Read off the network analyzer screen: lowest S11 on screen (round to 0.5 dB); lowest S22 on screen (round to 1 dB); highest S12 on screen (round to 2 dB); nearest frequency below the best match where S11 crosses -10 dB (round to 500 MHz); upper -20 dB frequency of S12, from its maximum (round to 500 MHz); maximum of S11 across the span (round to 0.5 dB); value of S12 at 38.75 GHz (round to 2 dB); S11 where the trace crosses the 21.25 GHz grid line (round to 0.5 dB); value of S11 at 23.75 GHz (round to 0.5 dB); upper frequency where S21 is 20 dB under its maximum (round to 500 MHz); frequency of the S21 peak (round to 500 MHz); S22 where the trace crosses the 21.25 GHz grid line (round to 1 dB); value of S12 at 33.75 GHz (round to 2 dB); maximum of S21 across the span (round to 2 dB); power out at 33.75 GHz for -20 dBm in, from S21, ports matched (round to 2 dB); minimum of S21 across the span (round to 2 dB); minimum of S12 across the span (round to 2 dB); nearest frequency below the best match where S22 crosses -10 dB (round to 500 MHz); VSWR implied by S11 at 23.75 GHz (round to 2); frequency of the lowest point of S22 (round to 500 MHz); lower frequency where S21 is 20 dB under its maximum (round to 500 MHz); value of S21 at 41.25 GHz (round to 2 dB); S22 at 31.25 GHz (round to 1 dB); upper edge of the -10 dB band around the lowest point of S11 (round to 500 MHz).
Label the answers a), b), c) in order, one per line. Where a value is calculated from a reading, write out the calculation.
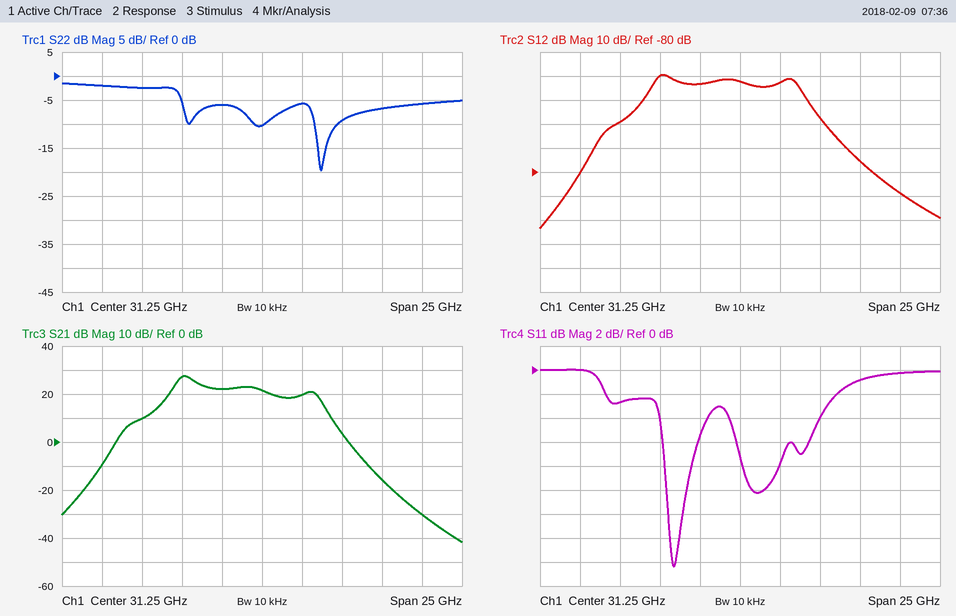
a) -16.5 dB
b) -20 dB
c) -40 dB
d) 26.5 GHz
e) 36.5 GHz
f) 0.0 dB
g) -76 dB
h) 0.0 dB
i) -2.5 dB
j) 36.0 GHz
k) 26.5 GHz
l) -2 dB
m) -42 dB
n) 28 dB
o) -20 dBm + (20 dB) = 0 dBm
p) -42 dB
q) -104 dB
r) 34.5 GHz
s) |Γ| = 10^(-2.5/20) = 0.7499; VSWR = (1 + 0.7499)/(1 − 0.7499) ≈ 7.00, so 6 to the nearest 2
t) 35.0 GHz
u) 23.0 GHz
v) -30 dB
w) -10 dB
x) 28.0 GHz
